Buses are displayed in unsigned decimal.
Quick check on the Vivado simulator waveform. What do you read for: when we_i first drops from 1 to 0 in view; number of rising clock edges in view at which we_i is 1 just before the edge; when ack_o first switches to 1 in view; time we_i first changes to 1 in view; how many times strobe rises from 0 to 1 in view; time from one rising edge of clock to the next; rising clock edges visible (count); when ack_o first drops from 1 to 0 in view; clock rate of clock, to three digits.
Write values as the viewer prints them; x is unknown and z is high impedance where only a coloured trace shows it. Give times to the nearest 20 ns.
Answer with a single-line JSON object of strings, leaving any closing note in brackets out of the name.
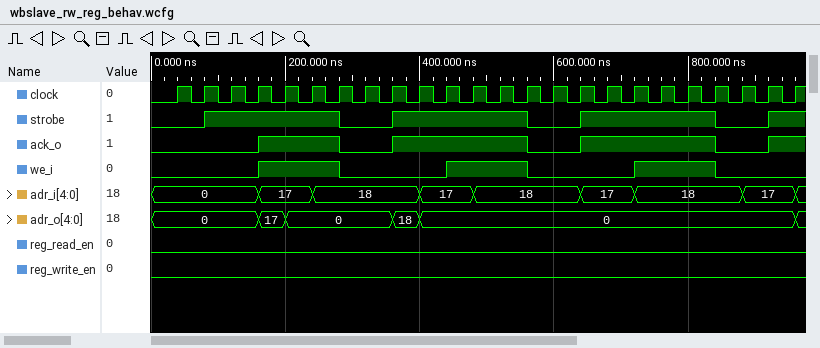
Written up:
{"when we_i first drops from 1 to 0 in view": "280 ns", "number of rising clock edges in view at which we_i is 1 just before the edge": "9", "when ack_o first switches to 1 in view": "160 ns", "time we_i first changes to 1 in view": "160 ns", "how many times strobe rises from 0 to 1 in view": "4", "time from one rising edge of clock to the next": "40 ns", "rising clock edges visible": "24", "when ack_o first drops from 1 to 0 in view": "280 ns", "clock rate of clock, to three digits": "25.0 MHz"}
